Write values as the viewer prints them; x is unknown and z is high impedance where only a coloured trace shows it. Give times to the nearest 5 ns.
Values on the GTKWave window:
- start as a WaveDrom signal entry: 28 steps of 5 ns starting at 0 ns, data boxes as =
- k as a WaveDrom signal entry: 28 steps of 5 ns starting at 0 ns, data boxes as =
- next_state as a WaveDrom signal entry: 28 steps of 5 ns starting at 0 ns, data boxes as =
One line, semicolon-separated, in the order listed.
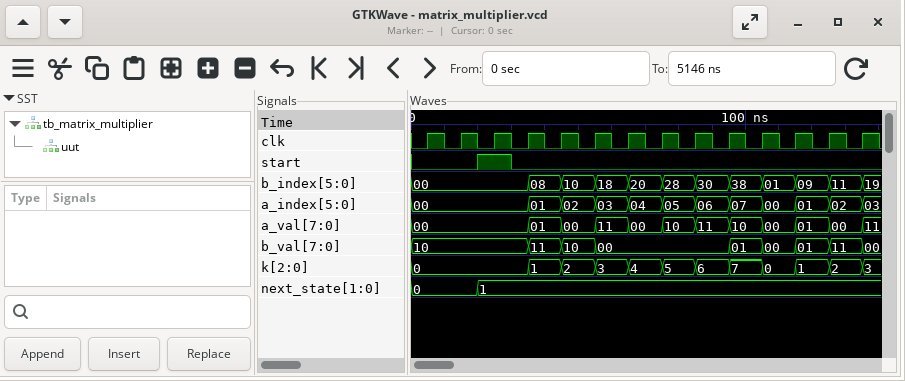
{name: 'start', wave: '0...1.0.....................'}; {name: 'k', wave: '=......=.=.=.=.=.=.=.=.=.=.=', data: '0 1 2 3 4 5 6 7 0 1 2 3'}; {name: 'next_state', wave: '=...=.......................', data: '0 1'}
